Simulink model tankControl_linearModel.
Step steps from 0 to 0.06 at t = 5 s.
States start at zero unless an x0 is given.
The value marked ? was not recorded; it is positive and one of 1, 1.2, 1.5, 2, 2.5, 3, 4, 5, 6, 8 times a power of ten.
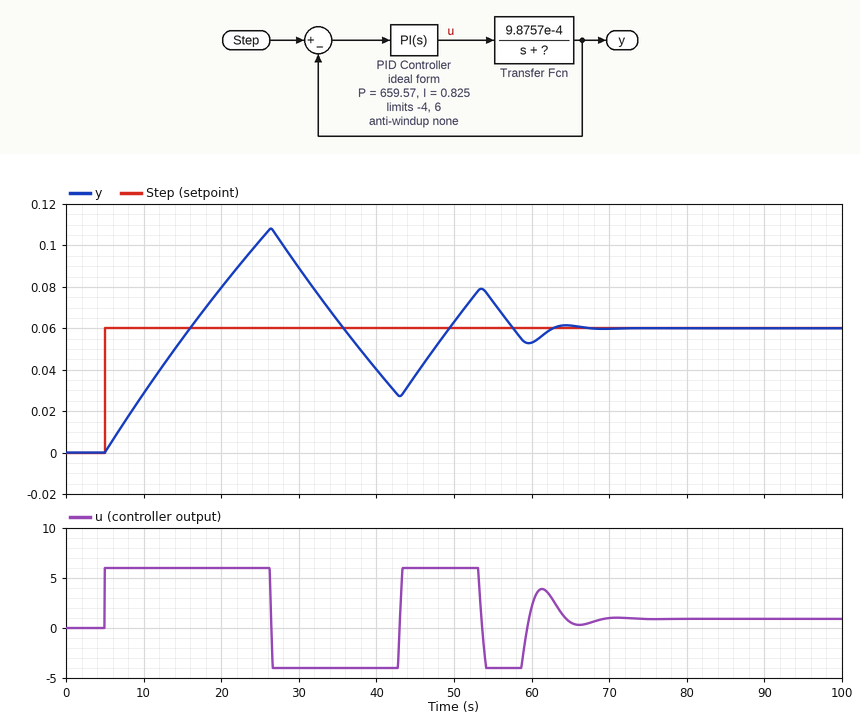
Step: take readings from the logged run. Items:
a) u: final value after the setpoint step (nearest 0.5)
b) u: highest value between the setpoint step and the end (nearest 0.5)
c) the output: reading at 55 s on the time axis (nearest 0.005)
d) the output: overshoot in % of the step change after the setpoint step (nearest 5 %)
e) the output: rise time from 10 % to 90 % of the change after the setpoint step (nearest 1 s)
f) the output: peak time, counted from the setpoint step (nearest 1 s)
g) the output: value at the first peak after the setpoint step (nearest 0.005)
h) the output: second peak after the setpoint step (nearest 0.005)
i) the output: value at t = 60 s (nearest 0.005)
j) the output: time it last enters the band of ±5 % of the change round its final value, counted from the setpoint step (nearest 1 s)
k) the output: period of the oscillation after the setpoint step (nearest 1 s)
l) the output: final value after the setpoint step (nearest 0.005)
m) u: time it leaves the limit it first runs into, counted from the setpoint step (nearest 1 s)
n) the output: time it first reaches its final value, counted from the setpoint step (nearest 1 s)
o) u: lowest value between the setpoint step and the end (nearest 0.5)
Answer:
1.0
6.0
0.075
80 %
9 s
21 s
0.110
0.080
0.055
57 s
27 s
0.060
21 s
11 s
-4.0
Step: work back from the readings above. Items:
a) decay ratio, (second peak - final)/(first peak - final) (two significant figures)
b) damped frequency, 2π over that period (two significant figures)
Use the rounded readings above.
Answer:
0.40
0.23 rad/s
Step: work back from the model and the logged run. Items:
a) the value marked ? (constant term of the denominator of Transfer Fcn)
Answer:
0.015
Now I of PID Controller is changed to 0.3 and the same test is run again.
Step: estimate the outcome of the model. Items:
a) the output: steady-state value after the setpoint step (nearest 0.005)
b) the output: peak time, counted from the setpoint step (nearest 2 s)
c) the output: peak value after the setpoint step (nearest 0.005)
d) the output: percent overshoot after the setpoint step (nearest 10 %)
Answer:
0.060
20 s
0.100
70 %
